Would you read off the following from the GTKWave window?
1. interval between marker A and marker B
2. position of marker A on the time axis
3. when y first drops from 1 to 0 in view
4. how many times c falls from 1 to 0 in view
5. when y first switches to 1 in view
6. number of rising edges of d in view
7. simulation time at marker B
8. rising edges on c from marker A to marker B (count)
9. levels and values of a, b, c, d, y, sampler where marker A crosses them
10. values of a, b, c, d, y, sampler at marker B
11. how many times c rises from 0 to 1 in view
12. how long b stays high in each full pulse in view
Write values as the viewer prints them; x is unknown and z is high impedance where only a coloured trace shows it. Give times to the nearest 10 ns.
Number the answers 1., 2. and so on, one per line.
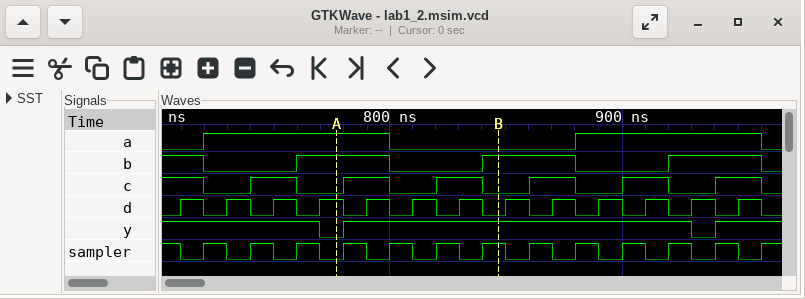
1. 70 ns
2. 780 ns
3. 770 ns
4. 7
5. 780 ns
6. 13
7. 850 ns
8. 2
9. a=1, b=1, c=0, d=1, y=0, sampler=0
10. a=0, b=1, c=0, d=0, y=1, sampler=1
11. 6
12. 40 ns, 40 ns, 40 ns
